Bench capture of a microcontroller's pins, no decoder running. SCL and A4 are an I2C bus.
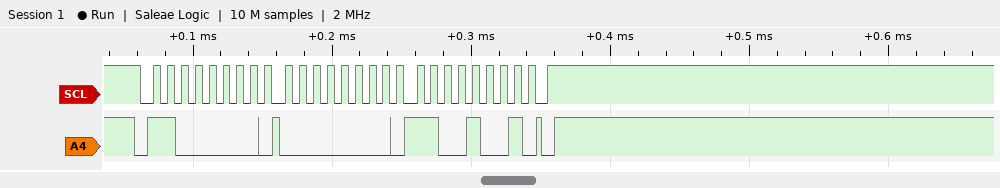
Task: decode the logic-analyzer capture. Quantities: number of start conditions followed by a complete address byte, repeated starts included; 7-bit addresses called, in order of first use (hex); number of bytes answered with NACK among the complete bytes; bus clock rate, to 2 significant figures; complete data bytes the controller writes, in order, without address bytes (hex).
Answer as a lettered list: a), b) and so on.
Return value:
a) 1
b) 0x60
c) 0
d) 100 kHz
e) 00 C9
